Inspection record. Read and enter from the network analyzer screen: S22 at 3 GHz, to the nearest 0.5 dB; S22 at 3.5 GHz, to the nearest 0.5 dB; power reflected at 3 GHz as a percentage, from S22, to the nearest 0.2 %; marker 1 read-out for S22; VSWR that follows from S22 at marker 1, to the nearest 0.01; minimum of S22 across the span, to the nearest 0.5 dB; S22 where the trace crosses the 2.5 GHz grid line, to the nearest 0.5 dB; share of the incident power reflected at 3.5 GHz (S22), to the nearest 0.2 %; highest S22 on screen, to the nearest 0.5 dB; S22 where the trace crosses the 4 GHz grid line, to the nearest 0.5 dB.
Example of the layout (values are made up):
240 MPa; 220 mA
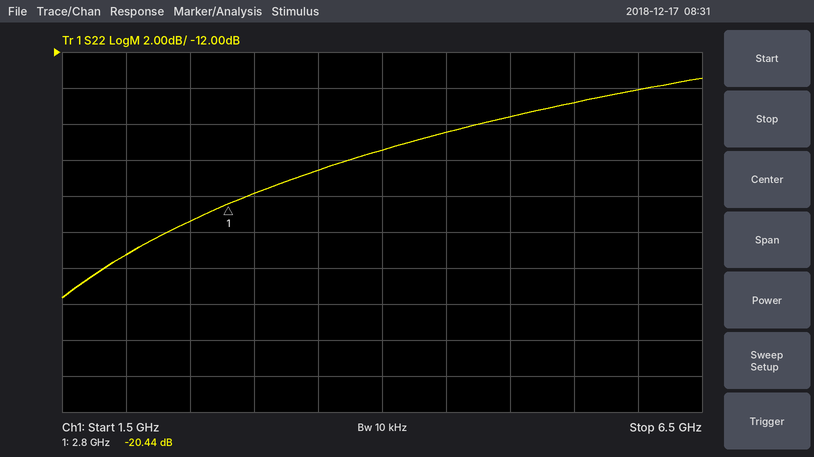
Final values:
-20.0 dB; -18.5 dB; 1.0 %; -20.44 dB; 1.21; -25.5 dB; -21.5 dB; 1.4 %; -13.5 dB; -17.5 dB
